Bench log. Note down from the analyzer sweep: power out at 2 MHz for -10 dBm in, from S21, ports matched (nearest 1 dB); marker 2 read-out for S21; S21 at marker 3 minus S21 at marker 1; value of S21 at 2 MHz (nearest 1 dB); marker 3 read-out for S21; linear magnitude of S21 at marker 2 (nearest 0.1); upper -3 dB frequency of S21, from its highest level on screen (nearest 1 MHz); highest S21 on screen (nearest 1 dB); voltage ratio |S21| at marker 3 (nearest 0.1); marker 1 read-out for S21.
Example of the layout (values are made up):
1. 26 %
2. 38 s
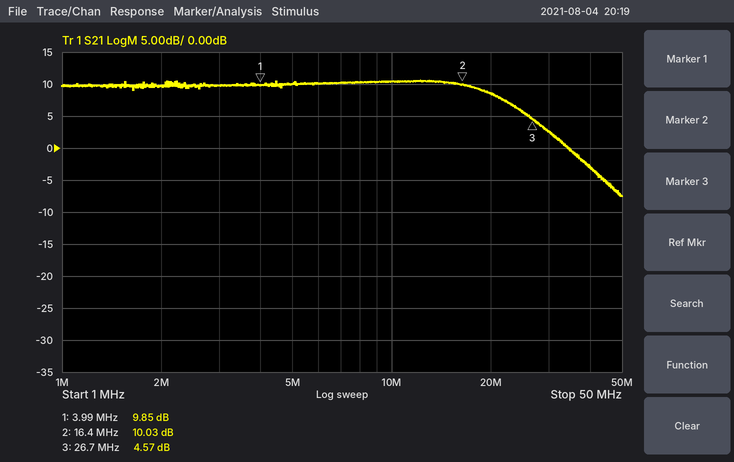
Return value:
1. 0 dBm
2. 10.03 dB
3. -5.28 dB
4. 10 dB
5. 4.57 dB
6. 3.2
7. 22 MHz
8. 11 dB
9. 1.7
10. 9.85 dB
